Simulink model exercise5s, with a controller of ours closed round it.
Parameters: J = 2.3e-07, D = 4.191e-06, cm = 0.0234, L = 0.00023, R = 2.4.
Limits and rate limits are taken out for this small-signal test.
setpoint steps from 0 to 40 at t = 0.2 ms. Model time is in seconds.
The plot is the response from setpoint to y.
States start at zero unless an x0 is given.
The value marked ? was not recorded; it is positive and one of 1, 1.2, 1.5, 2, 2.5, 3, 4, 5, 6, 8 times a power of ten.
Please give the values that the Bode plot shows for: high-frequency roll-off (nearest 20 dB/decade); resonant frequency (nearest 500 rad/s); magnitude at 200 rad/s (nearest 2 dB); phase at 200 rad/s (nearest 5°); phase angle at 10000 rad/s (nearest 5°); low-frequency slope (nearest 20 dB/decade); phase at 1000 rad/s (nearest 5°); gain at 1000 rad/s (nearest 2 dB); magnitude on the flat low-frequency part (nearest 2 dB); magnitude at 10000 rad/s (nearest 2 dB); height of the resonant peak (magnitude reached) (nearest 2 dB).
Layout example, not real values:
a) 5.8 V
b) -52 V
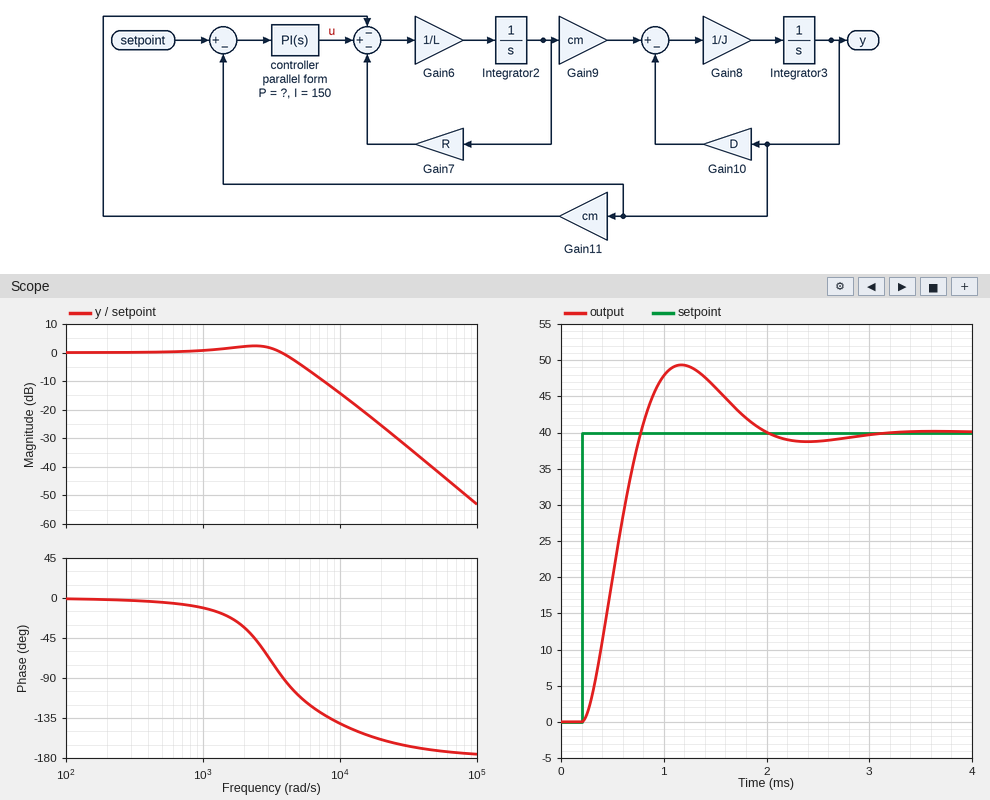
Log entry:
a) -40 dB/decade
b) 2500 rad/s
c) 0 dB
d) 0°
e) -140°
f) 0 dB/decade
g) -10°
h) 0 dB
i) 0 dB
j) -14 dB
k) 2 dB
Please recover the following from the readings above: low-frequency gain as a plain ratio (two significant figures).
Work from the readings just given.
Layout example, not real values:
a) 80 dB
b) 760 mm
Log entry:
a) 1.0
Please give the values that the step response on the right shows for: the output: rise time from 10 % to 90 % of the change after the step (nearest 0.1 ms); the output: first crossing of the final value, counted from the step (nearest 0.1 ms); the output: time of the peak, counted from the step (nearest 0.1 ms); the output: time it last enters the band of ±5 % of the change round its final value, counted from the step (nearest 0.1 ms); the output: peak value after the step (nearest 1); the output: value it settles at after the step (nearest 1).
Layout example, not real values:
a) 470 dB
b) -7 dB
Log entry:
a) 0.4 ms
b) 0.6 ms
c) 1.0 ms
d) 1.6 ms
e) 49
f) 40
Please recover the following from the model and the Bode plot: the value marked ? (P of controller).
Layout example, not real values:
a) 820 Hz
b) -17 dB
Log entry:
a) 0.05
